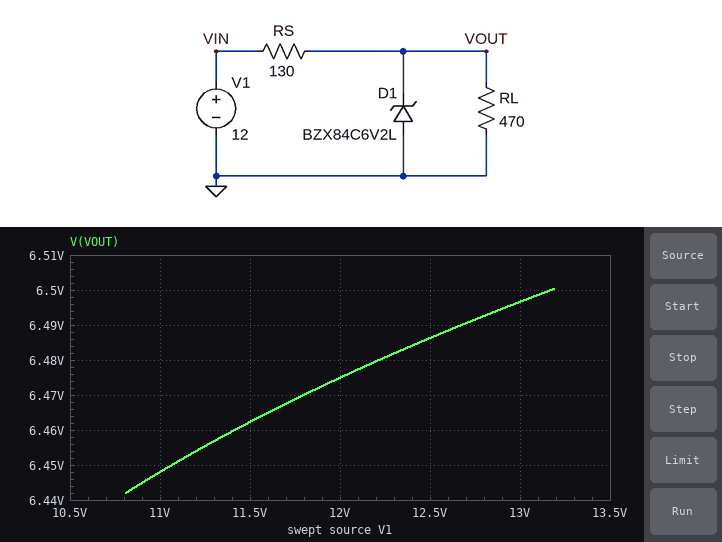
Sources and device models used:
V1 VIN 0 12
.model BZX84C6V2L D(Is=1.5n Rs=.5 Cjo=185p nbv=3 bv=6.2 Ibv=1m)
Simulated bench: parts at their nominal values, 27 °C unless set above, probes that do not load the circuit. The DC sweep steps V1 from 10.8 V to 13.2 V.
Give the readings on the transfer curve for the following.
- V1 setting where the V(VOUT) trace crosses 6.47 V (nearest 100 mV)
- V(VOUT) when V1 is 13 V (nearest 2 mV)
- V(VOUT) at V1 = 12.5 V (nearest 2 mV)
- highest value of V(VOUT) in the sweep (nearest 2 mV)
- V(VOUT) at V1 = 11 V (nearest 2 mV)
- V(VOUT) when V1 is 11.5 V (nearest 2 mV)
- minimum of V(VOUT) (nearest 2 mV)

11.8 V
6.496 V
6.486 V
6.500 V
6.448 V
6.462 V
6.442 V
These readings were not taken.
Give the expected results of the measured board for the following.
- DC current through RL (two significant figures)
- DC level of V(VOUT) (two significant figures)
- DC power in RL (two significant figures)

14 mA
6.5 V
89 mW
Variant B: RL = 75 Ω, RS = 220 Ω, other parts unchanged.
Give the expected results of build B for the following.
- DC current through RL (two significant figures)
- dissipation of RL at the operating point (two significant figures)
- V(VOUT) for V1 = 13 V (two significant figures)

41 mA
120 mW
3.3 V
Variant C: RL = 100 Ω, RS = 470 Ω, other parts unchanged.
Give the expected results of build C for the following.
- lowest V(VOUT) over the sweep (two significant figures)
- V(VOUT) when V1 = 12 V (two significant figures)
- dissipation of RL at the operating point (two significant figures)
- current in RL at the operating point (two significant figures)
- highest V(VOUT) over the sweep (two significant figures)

1.9 V
2.1 V
44 mW
21 mA
2.3 V
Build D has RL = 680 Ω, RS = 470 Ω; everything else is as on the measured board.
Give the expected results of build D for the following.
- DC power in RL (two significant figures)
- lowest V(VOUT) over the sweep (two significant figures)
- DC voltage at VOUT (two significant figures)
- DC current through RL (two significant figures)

58 mW
6.2 V
6.3 V
9.2 mA
